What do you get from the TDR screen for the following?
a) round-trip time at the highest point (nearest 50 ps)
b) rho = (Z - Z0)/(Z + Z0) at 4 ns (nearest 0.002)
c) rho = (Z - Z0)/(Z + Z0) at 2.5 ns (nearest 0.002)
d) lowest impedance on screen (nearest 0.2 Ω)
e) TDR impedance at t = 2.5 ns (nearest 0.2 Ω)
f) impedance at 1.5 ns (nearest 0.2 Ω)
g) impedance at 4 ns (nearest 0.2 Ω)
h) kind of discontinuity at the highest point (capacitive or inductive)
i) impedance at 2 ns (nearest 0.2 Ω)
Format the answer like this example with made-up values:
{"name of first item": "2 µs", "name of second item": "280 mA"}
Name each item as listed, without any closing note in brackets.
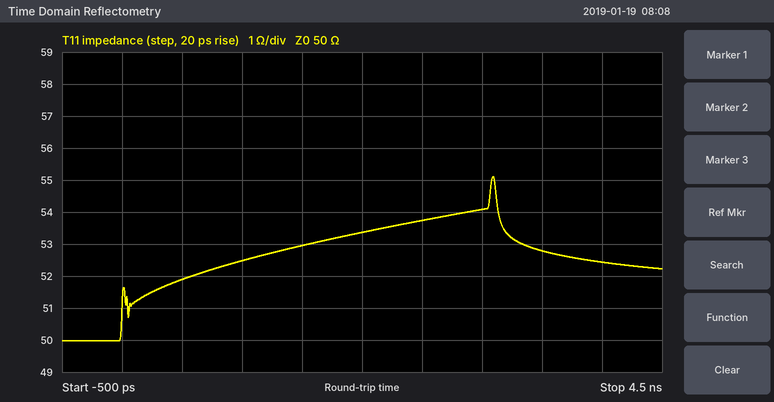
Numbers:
{"round-trip time at the highest point": "3.10 ns", "rho = (Z - Z0)/(Z + Z0) at 4 ns": "+0.024", "rho = (Z - Z0)/(Z + Z0) at 2.5 ns": "+0.036", "lowest impedance on screen": "50.0 Ω", "TDR impedance at t = 2.5 ns": "53.8 Ω", "impedance at 1.5 ns": "53.0 Ω", "impedance at 4 ns": "52.4 Ω", "kind of discontinuity at the highest point": "inductive", "impedance at 2 ns": "53.4 Ω"}
